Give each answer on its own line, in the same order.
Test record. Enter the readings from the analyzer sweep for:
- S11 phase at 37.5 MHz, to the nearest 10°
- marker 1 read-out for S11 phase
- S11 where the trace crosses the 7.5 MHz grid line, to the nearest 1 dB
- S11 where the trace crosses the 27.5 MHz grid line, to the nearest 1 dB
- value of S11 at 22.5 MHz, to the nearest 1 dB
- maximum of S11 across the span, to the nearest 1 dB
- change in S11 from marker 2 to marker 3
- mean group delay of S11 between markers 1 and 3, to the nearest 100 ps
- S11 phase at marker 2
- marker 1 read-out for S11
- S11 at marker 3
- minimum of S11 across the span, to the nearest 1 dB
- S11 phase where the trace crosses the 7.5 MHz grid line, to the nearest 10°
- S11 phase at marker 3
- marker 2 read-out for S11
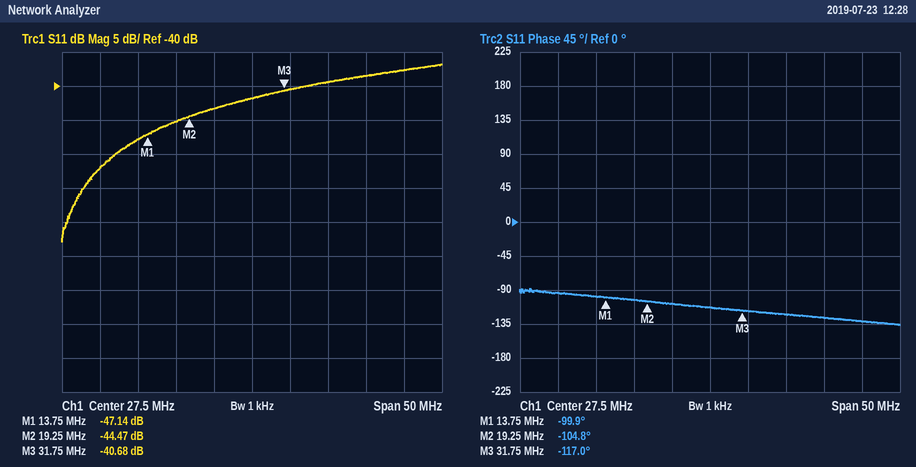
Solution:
-120°
-99.9°
-52 dB
-42 dB
-43 dB
-37 dB
3.79 dB
2.6 ns
-104.8°
-47.14 dB
-40.68 dB
-63 dB
-90°
-117.0°
-44.47 dB
